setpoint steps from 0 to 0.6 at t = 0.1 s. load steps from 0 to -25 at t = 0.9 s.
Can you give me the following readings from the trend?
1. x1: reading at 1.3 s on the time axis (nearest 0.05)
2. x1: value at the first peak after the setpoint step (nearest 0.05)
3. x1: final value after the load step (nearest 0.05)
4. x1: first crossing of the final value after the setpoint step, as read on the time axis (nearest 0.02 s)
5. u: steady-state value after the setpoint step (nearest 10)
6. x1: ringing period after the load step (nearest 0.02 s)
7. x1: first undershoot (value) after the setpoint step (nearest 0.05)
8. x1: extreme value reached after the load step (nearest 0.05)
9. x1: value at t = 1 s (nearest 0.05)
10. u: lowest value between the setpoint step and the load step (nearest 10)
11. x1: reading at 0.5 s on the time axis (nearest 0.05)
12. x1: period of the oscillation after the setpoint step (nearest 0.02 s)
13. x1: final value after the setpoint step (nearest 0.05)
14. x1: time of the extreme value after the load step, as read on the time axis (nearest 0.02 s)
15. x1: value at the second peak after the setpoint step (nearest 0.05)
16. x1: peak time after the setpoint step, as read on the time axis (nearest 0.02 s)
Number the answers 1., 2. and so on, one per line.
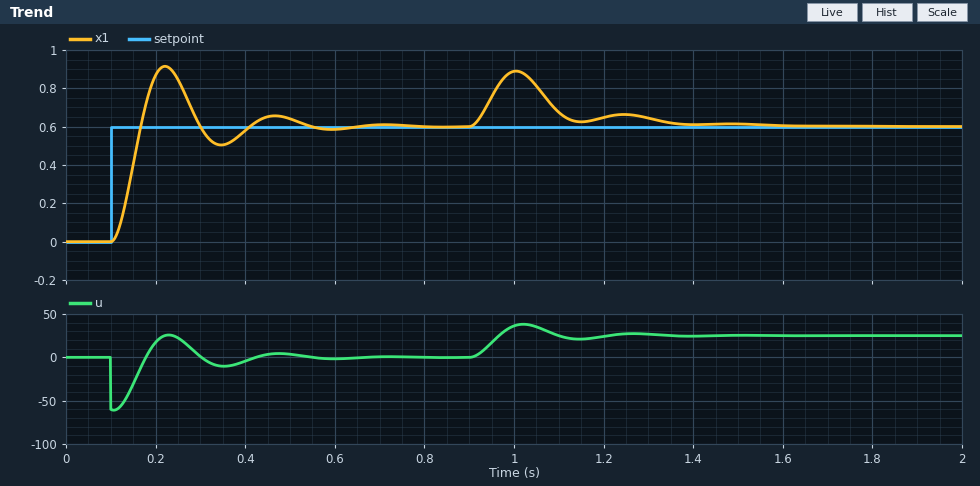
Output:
1. 0.65
2. 0.90
3. 0.60
4. 0.16 s
5. 0
6. 0.24 s
7. 0.50
8. 0.90
9. 0.90
10. -60
11. 0.65
12. 0.24 s
13. 0.60
14. 1.00 s
15. 0.65
16. 0.22 s
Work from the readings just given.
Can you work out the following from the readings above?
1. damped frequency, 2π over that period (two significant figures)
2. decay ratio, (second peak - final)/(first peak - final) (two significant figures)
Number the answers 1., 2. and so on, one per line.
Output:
1. 26 rad/s
2. 0.17
